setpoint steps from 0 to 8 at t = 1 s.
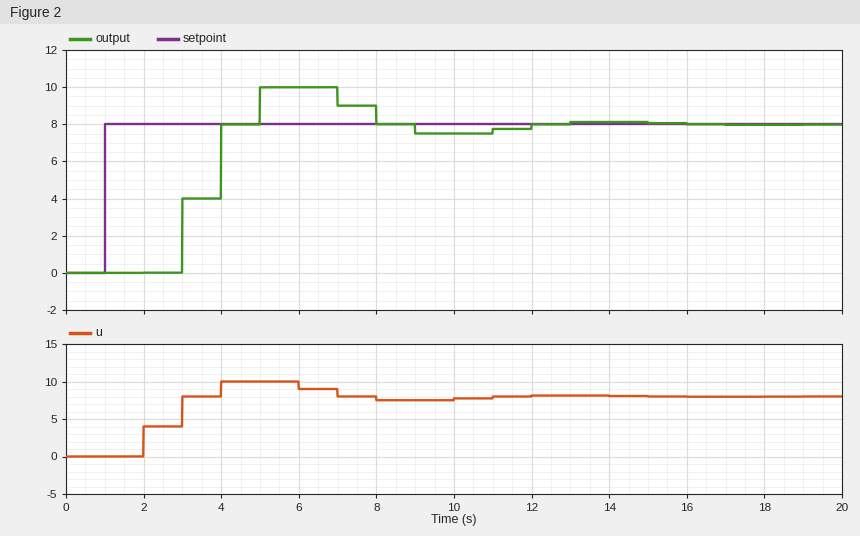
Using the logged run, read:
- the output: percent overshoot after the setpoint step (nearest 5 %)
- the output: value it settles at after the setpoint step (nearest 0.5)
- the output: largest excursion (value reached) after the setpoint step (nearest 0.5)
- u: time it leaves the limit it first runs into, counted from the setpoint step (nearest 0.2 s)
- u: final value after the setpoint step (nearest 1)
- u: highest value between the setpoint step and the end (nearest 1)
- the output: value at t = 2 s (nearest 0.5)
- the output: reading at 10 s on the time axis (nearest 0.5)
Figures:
25 %
8.0
10.0
1.0 s
8
10
0.0
7.5
